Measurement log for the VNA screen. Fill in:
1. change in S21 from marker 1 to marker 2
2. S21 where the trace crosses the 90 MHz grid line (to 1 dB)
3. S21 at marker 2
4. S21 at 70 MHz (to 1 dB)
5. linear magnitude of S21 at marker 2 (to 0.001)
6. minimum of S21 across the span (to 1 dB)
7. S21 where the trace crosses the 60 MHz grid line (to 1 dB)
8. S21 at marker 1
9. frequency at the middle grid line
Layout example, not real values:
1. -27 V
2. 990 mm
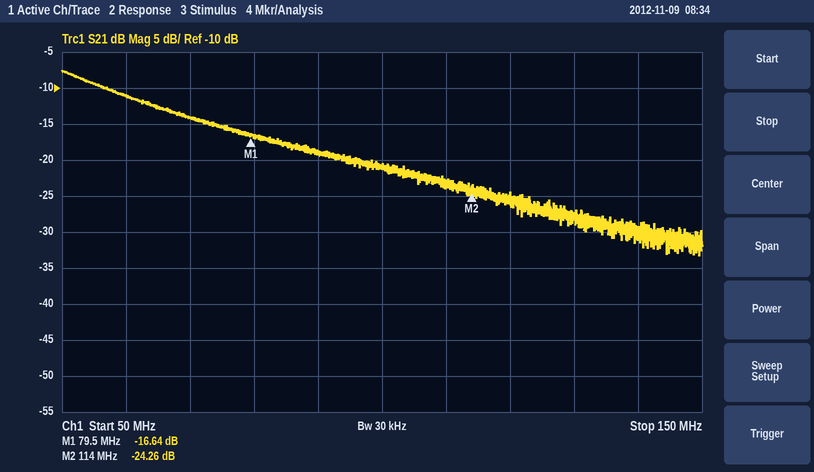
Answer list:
1. -7.62 dB
2. -19 dB
3. -24.26 dB
4. -14 dB
5. 0.061
6. -33 dB
7. -11 dB
8. -16.64 dB
9. 100 MHz
